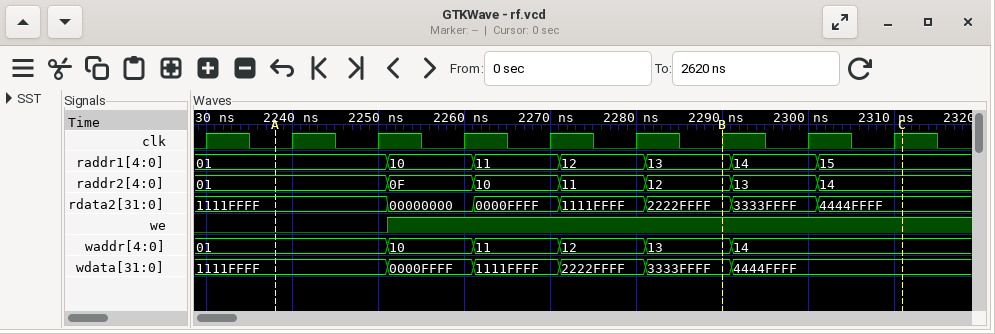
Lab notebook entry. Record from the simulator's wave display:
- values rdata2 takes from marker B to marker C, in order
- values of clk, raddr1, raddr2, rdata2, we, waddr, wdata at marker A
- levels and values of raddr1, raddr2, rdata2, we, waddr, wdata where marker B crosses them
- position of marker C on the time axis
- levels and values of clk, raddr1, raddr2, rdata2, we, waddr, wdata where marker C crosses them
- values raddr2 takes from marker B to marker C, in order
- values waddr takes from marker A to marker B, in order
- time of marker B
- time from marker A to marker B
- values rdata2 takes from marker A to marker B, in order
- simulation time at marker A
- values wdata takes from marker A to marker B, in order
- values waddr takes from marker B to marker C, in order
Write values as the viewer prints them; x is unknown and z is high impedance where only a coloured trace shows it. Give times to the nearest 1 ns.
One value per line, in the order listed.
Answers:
2222FFFF, 3333FFFF, 4444FFFF
clk=0, raddr1=01, raddr2=01, rdata2=1111FFFF, we=0, waddr=01, wdata=1111FFFF
raddr1=13, raddr2=12, rdata2=2222FFFF, we=1, waddr=13, wdata=3333FFFF
2311 ns
clk=1, raddr1=15, raddr2=14, rdata2=4444FFFF, we=1, waddr=14, wdata=4444FFFF
12, 13, 14
01, 10, 11, 12, 13
2290 ns
52 ns
1111FFFF, 00000000, 0000FFFF, 1111FFFF, 2222FFFF
2238 ns
1111FFFF, 0000FFFF, 1111FFFF, 2222FFFF, 3333FFFF
13, 14
